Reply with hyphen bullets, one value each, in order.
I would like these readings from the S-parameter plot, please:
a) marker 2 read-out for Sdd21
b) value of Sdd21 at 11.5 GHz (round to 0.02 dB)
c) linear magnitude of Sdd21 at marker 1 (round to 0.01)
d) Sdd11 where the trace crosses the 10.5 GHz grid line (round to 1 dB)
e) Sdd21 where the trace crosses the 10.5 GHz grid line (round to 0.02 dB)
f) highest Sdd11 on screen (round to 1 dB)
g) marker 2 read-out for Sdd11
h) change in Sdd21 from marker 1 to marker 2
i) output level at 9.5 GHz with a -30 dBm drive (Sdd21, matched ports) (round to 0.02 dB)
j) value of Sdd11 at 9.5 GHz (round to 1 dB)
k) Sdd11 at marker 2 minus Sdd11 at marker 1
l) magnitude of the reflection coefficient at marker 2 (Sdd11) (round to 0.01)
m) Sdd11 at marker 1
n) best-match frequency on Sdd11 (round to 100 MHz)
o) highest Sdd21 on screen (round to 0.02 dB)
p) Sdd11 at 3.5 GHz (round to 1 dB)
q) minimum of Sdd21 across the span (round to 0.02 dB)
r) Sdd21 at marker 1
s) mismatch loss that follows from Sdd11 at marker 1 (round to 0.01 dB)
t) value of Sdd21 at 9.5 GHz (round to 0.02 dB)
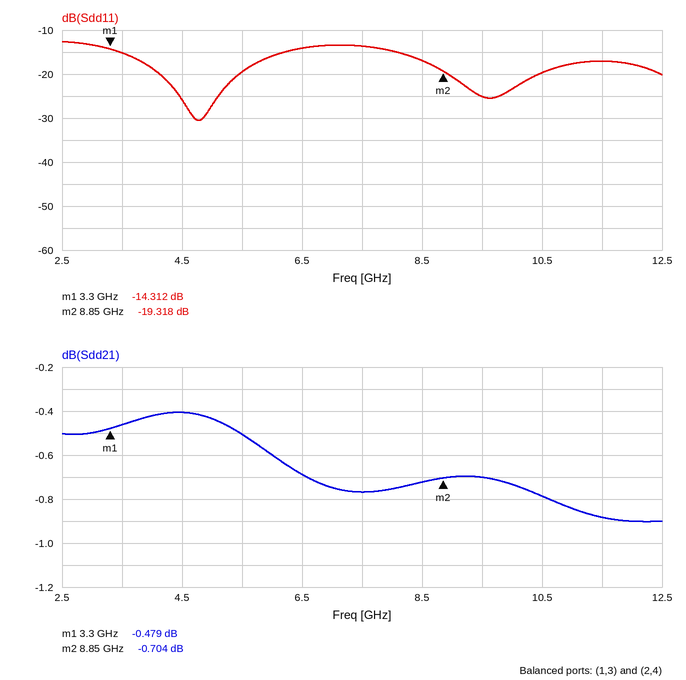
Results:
- -0.704 dB
- -0.88 dB
- 0.95
- -20 dB
- -0.78 dB
- -13 dB
- -19.318 dB
- -0.225 dB
- -30.70 dBm
- -25 dB
- -5.006 dB
- 0.11
- -14.312 dB
- 4.8 GHz
- -0.40 dB
- -15 dB
- -0.90 dB
- -0.479 dB
- 0.16 dB
- -0.70 dB
